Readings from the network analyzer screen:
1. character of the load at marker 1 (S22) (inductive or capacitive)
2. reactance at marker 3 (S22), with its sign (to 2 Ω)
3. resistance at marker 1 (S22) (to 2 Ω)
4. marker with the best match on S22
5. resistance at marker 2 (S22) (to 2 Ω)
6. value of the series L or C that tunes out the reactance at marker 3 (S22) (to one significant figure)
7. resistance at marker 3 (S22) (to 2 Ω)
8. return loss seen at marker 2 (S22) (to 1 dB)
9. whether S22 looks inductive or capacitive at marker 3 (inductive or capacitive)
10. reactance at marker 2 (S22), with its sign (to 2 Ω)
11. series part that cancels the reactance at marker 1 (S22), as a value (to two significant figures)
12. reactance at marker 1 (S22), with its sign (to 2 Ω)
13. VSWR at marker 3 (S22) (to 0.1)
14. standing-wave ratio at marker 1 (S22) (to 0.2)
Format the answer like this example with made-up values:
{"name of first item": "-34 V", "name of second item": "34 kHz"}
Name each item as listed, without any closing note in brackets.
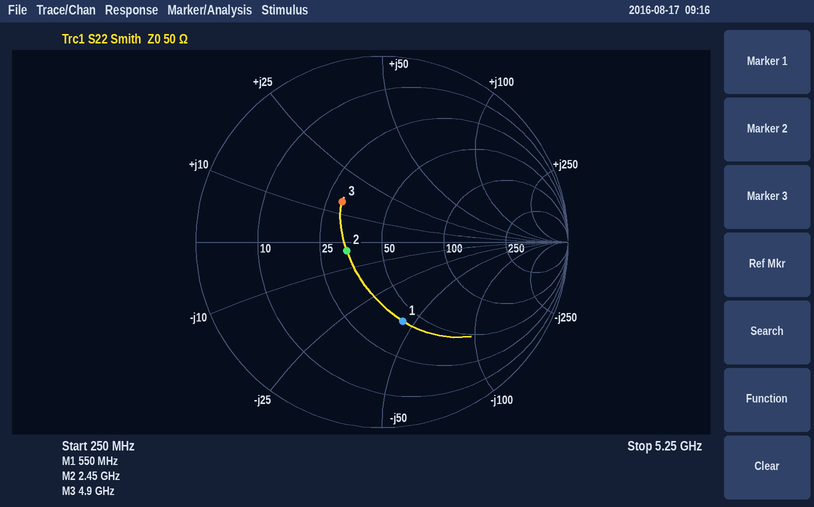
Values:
{"character of the load at marker 1 (S22)": "capacitive", "reactance at marker 3 (S22), with its sign": "+14 Ω", "resistance at marker 1 (S22)": "42 Ω", "marker with the best match on S22": "marker 2", "resistance at marker 2 (S22)": "34 Ω", "value of the series L or C that tunes out the reactance at marker 3 (S22)": "2 pF", "resistance at marker 3 (S22)": "30 Ω", "return loss seen at marker 2 (S22)": "14 dB", "whether S22 looks inductive or capacitive at marker 3": "inductive", "reactance at marker 2 (S22), with its sign": "-4 Ω", "series part that cancels the reactance at marker 1 (S22), as a value": "13 nH", "reactance at marker 1 (S22), with its sign": "-44 Ω", "VSWR at marker 3 (S22)": "1.9", "standing-wave ratio at marker 1 (S22)": "2.6"}
